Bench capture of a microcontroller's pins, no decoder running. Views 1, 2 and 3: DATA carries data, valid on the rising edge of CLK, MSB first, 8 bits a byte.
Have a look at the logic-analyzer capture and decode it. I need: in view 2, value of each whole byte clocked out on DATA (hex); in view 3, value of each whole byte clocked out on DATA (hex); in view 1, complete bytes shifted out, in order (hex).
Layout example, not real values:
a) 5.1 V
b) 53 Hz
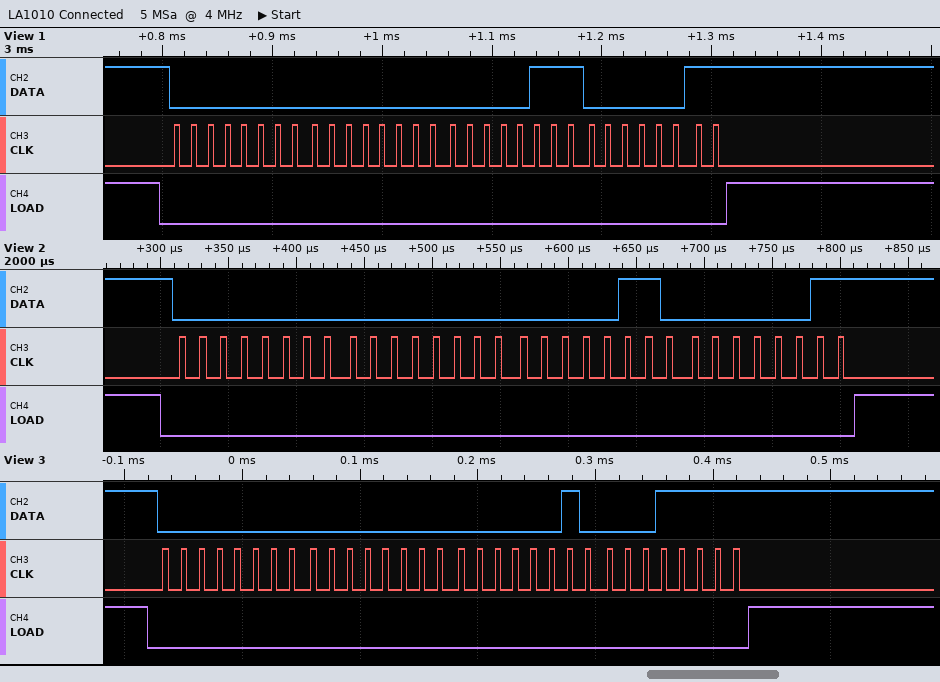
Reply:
a) 0x00 0x00 0x06 0x03
b) 00 00 02 1F
c) 00 00 07 03
